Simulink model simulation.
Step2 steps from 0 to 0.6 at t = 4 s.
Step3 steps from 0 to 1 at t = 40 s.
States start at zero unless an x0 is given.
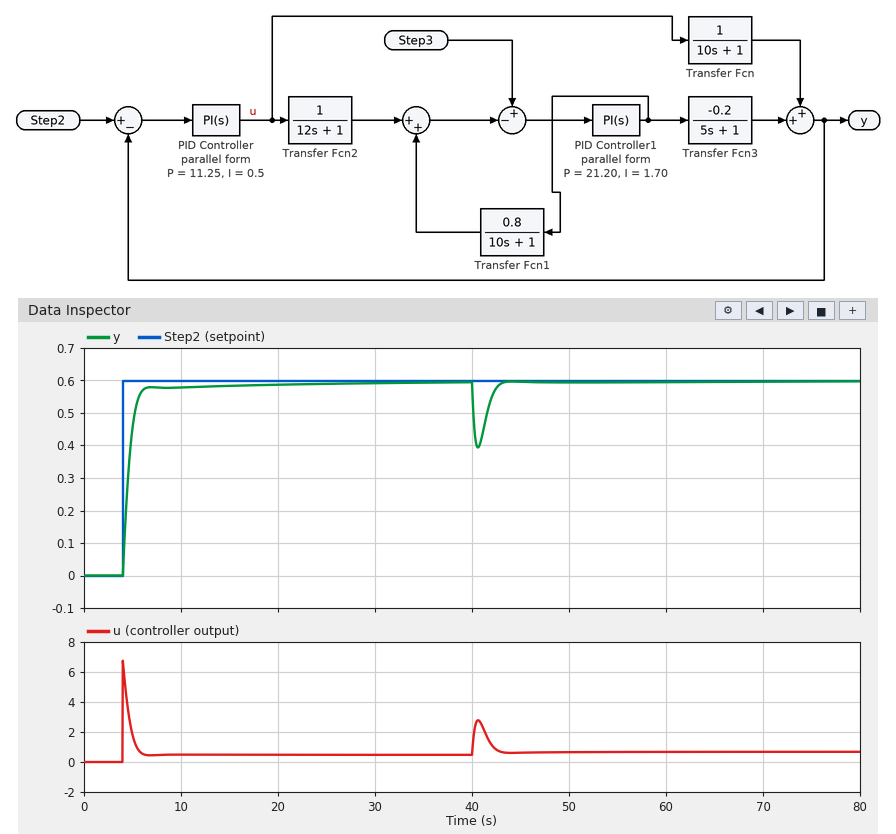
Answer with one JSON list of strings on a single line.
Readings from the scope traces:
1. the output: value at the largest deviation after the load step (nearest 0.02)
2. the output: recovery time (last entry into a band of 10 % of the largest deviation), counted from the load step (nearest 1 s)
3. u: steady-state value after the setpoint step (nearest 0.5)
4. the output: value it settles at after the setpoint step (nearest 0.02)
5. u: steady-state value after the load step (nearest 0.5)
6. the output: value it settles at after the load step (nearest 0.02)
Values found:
["0.40", "3 s", "0.5", "0.60", "0.5", "0.60"]
